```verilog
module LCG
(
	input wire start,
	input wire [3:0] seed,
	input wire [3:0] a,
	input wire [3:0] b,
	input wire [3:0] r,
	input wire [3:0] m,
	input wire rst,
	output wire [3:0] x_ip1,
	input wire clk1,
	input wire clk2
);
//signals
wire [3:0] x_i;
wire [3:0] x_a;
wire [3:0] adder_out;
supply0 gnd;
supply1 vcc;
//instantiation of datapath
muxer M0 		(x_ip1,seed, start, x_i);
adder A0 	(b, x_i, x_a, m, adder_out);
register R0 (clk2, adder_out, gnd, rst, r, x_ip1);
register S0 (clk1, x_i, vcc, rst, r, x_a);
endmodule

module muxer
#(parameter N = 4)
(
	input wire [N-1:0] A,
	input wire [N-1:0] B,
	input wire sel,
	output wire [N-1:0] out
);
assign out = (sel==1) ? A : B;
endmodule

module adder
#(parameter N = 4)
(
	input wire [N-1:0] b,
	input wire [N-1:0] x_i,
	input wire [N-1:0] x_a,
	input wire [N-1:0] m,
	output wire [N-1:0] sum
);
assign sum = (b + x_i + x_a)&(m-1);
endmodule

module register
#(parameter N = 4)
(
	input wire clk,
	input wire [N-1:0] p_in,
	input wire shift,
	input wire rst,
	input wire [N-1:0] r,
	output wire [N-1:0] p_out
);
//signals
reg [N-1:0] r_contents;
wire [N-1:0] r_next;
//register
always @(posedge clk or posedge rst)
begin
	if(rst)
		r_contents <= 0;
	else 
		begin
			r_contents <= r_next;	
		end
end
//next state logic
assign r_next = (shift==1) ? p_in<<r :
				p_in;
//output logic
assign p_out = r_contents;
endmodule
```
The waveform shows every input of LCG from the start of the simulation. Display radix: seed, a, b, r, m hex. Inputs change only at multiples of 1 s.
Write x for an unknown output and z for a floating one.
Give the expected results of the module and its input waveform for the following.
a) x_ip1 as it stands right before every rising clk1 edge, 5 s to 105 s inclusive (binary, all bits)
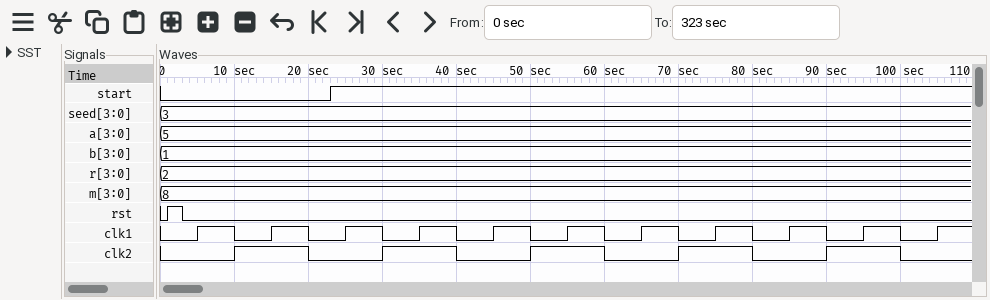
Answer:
0000, 0000, 0000, 0001, 0001, 0110, 0110, 0111, 0111, 0100, 0100
